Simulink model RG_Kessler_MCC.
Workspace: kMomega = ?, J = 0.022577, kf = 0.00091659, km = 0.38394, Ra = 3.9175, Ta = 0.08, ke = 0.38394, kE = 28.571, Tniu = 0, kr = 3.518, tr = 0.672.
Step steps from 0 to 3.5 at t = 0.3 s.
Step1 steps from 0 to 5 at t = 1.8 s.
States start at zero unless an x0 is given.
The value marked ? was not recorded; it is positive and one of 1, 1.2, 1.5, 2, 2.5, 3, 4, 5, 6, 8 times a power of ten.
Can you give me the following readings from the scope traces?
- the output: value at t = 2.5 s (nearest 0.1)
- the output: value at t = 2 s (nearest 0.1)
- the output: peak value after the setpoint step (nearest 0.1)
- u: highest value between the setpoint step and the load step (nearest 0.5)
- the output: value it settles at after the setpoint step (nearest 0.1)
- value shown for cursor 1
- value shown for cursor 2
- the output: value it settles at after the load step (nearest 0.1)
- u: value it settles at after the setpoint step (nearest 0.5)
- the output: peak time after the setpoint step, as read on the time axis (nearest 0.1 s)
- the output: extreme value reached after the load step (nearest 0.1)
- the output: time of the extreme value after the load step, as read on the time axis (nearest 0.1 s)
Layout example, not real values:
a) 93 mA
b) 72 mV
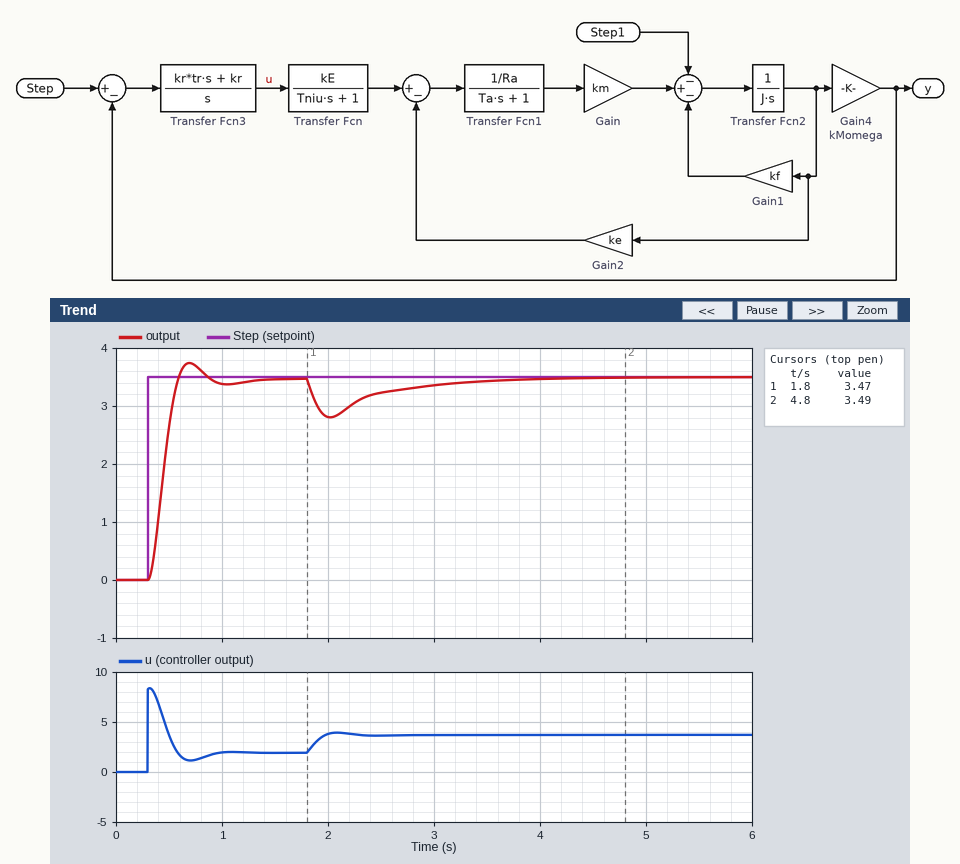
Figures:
a) 3.2
b) 2.8
c) 3.7
d) 8.5
e) 3.5
f) 3.47
g) 3.49
h) 3.5
i) 2.0
j) 0.7 s
k) 2.8
l) 2.0 s
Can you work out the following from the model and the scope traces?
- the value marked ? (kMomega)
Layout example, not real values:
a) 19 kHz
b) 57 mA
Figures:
a) 0.025
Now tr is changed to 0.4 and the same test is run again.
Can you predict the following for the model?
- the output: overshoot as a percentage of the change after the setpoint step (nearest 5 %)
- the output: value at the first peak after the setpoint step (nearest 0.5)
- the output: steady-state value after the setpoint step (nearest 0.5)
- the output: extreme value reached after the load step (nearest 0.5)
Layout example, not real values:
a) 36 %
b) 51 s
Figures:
a) 10 %
b) 4.0
c) 3.5
d) 2.5
